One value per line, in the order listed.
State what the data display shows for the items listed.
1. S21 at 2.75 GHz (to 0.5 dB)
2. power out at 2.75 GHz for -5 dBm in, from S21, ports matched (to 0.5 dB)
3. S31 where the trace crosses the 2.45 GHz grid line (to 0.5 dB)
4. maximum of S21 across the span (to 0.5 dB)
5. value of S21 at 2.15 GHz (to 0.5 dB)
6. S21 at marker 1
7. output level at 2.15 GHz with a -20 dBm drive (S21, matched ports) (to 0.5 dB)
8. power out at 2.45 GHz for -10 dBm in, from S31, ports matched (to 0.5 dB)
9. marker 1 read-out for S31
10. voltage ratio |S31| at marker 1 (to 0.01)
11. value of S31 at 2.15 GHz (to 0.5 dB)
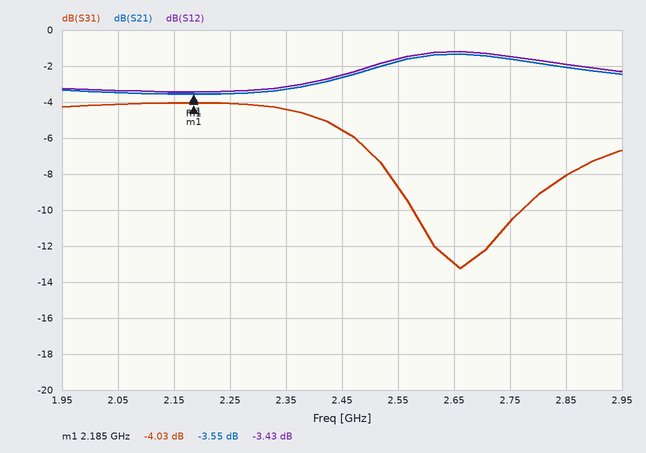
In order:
-1.5 dB
-6.5 dBm
-5.5 dB
-1.5 dB
-3.5 dB
-3.55 dB
-23.5 dBm
-15.5 dBm
-4.03 dB
0.63
-4.0 dB
